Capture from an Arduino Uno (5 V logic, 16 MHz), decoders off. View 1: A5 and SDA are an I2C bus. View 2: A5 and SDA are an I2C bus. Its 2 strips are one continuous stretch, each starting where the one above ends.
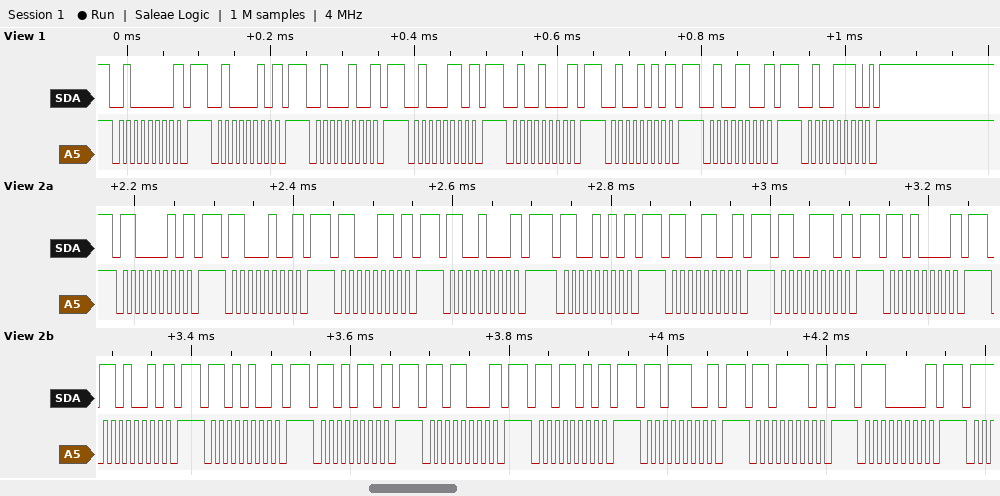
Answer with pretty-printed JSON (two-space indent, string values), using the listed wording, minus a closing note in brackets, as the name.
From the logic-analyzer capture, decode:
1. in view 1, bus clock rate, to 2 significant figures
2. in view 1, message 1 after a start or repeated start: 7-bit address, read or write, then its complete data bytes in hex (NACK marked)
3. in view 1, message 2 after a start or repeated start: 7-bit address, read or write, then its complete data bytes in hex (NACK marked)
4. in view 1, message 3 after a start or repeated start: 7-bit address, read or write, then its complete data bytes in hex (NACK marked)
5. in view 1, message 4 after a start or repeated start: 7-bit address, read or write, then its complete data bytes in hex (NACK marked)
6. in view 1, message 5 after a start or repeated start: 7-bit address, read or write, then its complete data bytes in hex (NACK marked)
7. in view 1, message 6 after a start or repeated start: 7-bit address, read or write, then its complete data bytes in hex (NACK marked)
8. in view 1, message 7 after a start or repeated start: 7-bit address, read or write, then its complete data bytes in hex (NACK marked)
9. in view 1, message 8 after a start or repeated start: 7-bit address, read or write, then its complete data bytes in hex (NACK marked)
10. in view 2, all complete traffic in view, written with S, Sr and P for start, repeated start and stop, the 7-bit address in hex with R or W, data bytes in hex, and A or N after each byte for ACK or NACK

{
  "in view 1, bus clock rate, to 2 significant figures": "100 kHz",
  "in view 1, message 1 after a start or repeated start: 7-bit address, read or write, then its complete data bytes in hex": "0x20 write NACK",
  "in view 1, message 2 after a start or repeated start: 7-bit address, read or write, then its complete data bytes in hex": "0x21 write NACK",
  "in view 1, message 3 after a start or repeated start: 7-bit address, read or write, then its complete data bytes in hex": "0x22 write NACK",
  "in view 1, message 4 after a start or repeated start: 7-bit address, read or write, then its complete data bytes in hex": "0x23 write NACK",
  "in view 1, message 5 after a start or repeated start: 7-bit address, read or write, then its complete data bytes in hex": "0x24 write NACK",
  "in view 1, message 6 after a start or repeated start: 7-bit address, read or write, then its complete data bytes in hex": "0x25 write NACK",
  "in view 1, message 7 after a start or repeated start: 7-bit address, read or write, then its complete data bytes in hex": "0x26 write NACK",
  "in view 1, message 8 after a start or repeated start: 7-bit address, read or write, then its complete data bytes in hex": "0x27 write",
  "in view 2, all complete traffic in view, written with S, Sr and P for start, repeated start and stop, the 7-bit address in hex with R or W, data bytes in hex, and A or N after each byte for ACK or NACK": "S 61W N P S 62W N P S 63W N P S 64W N P S 65W N P S 66W N P S 67W N P S 68W N P S 69W N P S 6AW N P S 6BW N P S 6CW N P S 6DW N P S 6EW N P S 6FW N P S 70W N P"
}
